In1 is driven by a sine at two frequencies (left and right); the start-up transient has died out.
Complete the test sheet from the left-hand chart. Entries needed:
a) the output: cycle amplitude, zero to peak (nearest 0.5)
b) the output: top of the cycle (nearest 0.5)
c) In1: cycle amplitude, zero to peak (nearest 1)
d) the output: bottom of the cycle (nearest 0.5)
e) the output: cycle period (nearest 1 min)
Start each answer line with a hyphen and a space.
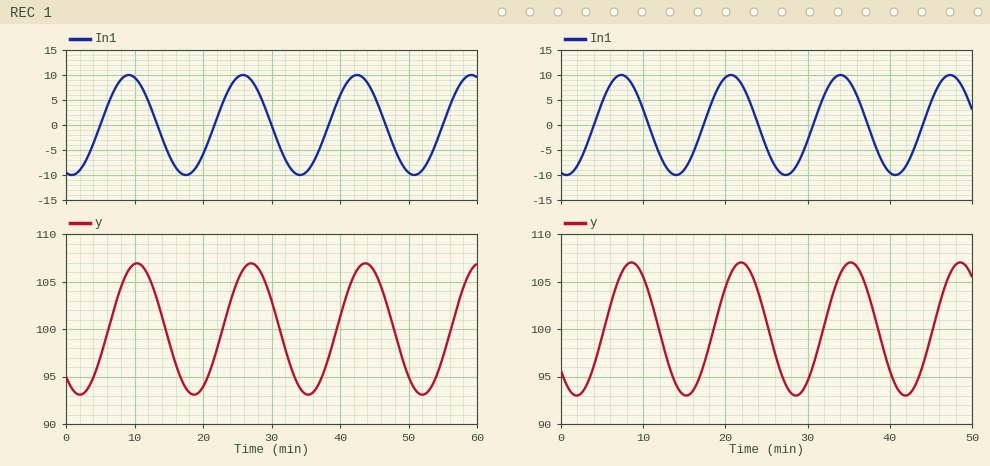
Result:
- 7.0
- 107.0
- 10
- 93.0
- 17 min
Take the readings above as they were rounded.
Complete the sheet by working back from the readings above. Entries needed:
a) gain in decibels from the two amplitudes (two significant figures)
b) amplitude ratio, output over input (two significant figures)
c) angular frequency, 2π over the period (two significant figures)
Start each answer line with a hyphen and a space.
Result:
- -3.1 dB
- 0.70
- 0.37 rad/min
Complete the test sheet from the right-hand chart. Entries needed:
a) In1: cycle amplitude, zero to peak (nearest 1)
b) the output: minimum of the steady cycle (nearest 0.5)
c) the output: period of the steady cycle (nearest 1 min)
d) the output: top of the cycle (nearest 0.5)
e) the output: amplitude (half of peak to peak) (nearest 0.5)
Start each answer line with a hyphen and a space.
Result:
- 10
- 93.0
- 13 min
- 107.0
- 7.0
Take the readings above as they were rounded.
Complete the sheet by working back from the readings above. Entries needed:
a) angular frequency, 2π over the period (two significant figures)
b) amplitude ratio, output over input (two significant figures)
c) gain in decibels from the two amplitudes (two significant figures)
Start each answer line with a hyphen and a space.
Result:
- 0.48 rad/min
- 0.70
- -3.1 dB
